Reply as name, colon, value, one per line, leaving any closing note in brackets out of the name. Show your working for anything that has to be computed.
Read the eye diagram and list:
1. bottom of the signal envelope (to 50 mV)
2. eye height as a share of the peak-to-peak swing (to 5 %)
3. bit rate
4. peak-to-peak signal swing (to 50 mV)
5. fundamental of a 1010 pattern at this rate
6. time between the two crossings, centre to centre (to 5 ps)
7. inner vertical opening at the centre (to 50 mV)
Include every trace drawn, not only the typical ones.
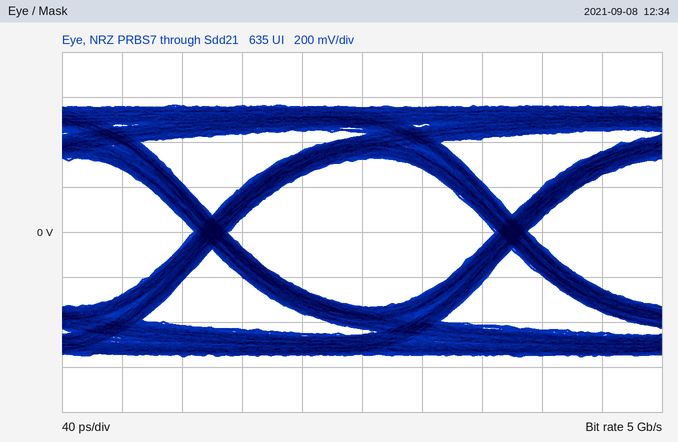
bottom of the signal envelope: -550 mV
eye height as a share of the peak-to-peak swing: 650 mV / 1.10 V ≈ 59.1 %, so 60 % to the nearest 5 %
bit rate: 5 Gb/s
peak-to-peak signal swing: 1.10 V
fundamental of a 1010 pattern at this rate: 2.5 GHz
time between the two crossings, centre to centre: 200 ps
inner vertical opening at the centre: 650 mV
